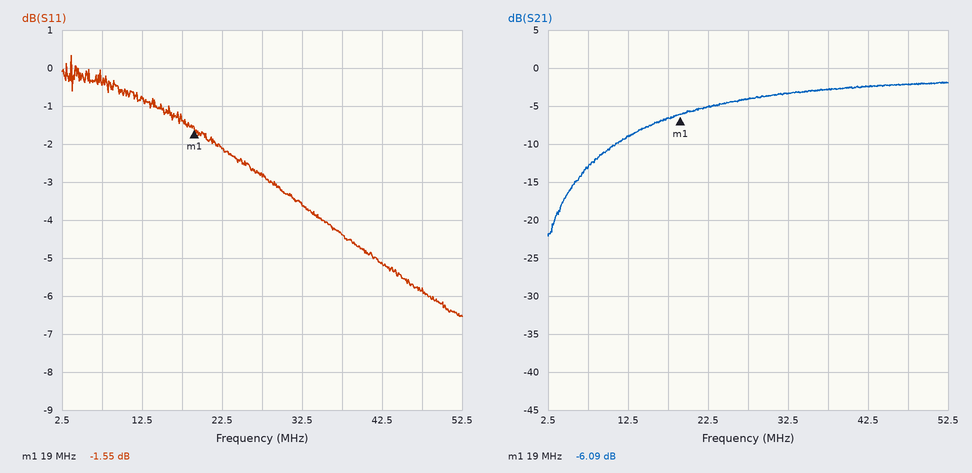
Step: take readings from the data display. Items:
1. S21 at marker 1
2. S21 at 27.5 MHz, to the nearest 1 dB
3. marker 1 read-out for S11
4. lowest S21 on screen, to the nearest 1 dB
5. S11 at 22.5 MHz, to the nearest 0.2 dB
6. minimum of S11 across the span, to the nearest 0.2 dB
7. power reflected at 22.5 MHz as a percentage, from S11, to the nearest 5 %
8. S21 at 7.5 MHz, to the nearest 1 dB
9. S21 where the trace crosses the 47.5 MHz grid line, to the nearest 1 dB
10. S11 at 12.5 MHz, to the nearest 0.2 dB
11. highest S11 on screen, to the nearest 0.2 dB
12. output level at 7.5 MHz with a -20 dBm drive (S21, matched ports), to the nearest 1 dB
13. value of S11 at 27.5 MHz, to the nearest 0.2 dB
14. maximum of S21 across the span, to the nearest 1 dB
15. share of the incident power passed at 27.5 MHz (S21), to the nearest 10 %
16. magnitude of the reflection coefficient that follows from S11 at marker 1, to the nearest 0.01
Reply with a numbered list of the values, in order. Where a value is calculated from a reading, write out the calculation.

1. -6.09 dB
2. -4 dB
3. -1.55 dB
4. -22 dB
5. -2.2 dB
6. -6.6 dB
7. 10^(-2.2/10) ≈ 60 %
8. -13 dB
9. -2 dB
10. -0.8 dB
11. 0.4 dB
12. -20 dBm + (-13 dB) = -33 dBm
13. -2.8 dB
14. -2 dB
15. 10^(-4/10) ≈ 40 %
16. 10^(-1.55/20) ≈ 0.84
